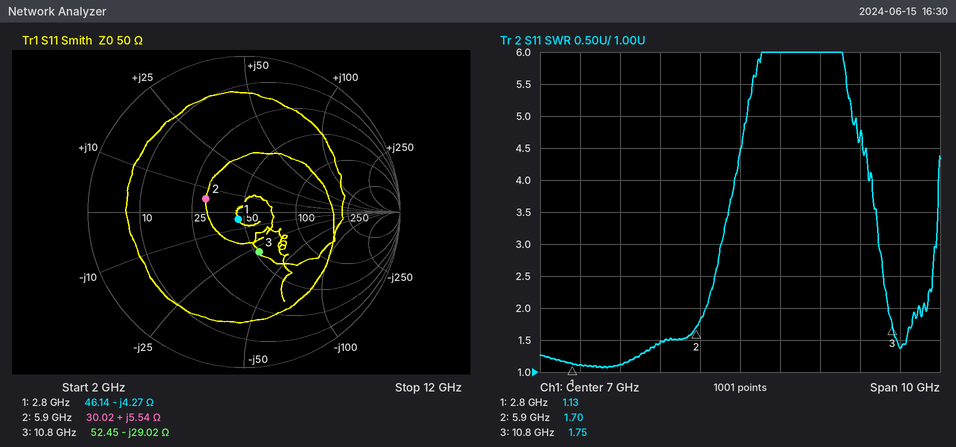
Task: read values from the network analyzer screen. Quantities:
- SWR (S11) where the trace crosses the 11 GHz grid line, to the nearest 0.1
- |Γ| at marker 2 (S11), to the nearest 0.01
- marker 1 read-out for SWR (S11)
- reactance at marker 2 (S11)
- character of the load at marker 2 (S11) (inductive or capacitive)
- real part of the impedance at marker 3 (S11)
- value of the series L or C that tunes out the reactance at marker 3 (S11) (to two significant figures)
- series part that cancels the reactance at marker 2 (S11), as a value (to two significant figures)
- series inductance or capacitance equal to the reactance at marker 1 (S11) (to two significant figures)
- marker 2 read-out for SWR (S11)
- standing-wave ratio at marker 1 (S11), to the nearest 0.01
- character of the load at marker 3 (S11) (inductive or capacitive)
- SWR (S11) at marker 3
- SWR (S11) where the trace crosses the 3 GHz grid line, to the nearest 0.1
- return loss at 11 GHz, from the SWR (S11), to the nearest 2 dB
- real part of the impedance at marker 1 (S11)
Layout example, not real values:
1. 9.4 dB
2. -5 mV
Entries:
1. 1.4
2. 0.26
3. 1.13
4. +5.54 Ω
5. inductive
6. 52.45 Ω
7. 430 pH
8. 4.9 pF
9. 13 pF
10. 1.70
11. 1.13
12. capacitive
13. 1.75
14. 1.1
15. 16 dB
16. 46.14 Ω
